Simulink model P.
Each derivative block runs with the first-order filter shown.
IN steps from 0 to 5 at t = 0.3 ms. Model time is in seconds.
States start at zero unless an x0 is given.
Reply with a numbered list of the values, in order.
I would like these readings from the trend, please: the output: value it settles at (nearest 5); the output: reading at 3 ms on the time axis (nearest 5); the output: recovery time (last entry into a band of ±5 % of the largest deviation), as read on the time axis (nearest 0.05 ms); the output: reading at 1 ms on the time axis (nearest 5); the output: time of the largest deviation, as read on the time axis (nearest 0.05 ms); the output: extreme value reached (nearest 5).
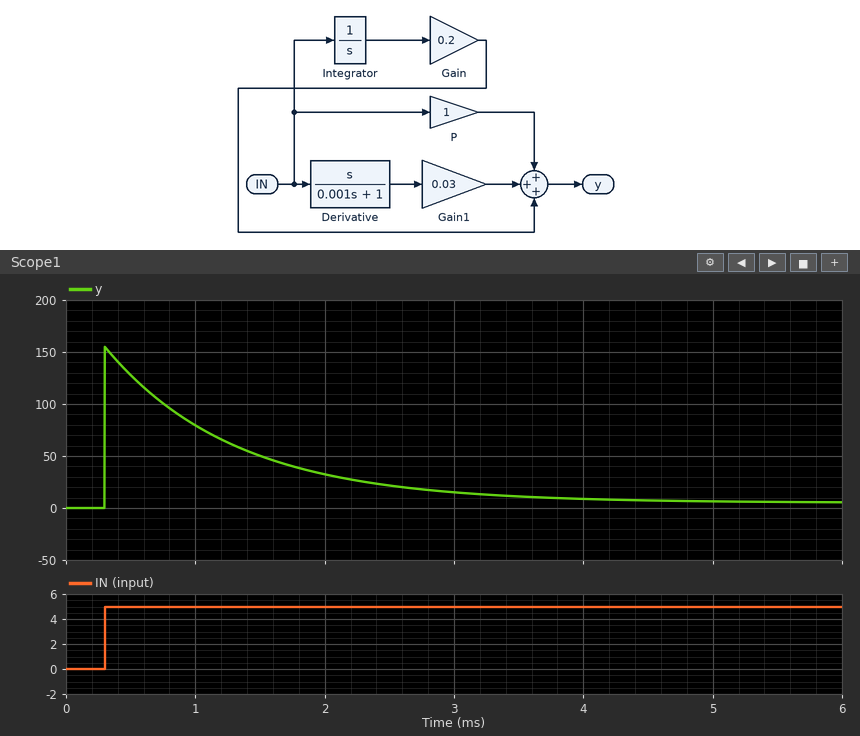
1. 5
2. 15
3. 3.25 ms
4. 80
5. 0.30 ms
6. 155
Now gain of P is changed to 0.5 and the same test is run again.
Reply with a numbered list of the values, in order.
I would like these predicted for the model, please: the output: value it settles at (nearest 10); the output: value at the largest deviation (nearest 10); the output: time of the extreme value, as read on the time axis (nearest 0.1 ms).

1. 0
2. 150
3. 0.3 ms
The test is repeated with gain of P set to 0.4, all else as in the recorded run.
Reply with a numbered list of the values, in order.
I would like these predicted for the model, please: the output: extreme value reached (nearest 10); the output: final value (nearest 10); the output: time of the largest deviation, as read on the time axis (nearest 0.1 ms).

1. 150
2. 0
3. 0.3 ms
